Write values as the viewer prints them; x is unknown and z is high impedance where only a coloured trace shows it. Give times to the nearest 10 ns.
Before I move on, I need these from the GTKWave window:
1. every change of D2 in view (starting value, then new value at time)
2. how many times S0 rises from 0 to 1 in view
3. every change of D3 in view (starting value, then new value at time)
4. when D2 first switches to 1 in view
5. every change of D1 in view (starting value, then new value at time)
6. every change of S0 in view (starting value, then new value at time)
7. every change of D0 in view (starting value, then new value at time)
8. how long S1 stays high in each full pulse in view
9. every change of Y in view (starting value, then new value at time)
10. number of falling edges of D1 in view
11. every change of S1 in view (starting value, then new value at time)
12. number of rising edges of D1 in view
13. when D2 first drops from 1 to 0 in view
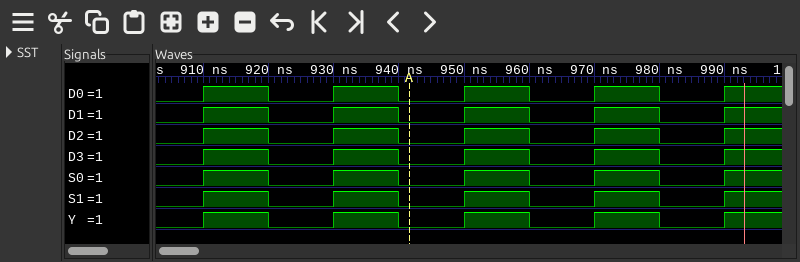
0, 1 at 910 ns, 0 at 920 ns, 1 at 930 ns, 0 at 940 ns, 1 at 950 ns, 0 at 960 ns, 1 at 970 ns, 0 at 980 ns, 1 at 990 ns
5
0, 1 at 910 ns, 0 at 920 ns, 1 at 930 ns, 0 at 940 ns, 1 at 950 ns, 0 at 960 ns, 1 at 970 ns, 0 at 980 ns, 1 at 990 ns
910 ns
0, 1 at 910 ns, 0 at 920 ns, 1 at 930 ns, 0 at 940 ns, 1 at 950 ns, 0 at 960 ns, 1 at 970 ns, 0 at 980 ns, 1 at 990 ns
0, 1 at 910 ns, 0 at 920 ns, 1 at 930 ns, 0 at 940 ns, 1 at 950 ns, 0 at 960 ns, 1 at 970 ns, 0 at 980 ns, 1 at 990 ns
0, 1 at 910 ns, 0 at 920 ns, 1 at 930 ns, 0 at 940 ns, 1 at 950 ns, 0 at 960 ns, 1 at 970 ns, 0 at 980 ns, 1 at 990 ns
10 ns, 10 ns, 10 ns, 10 ns
0, 1 at 910 ns, 0 at 920 ns, 1 at 930 ns, 0 at 940 ns, 1 at 950 ns, 0 at 960 ns, 1 at 970 ns, 0 at 980 ns, 1 at 990 ns
4
0, 1 at 910 ns, 0 at 920 ns, 1 at 930 ns, 0 at 940 ns, 1 at 950 ns, 0 at 960 ns, 1 at 970 ns, 0 at 980 ns, 1 at 990 ns
5
920 ns
